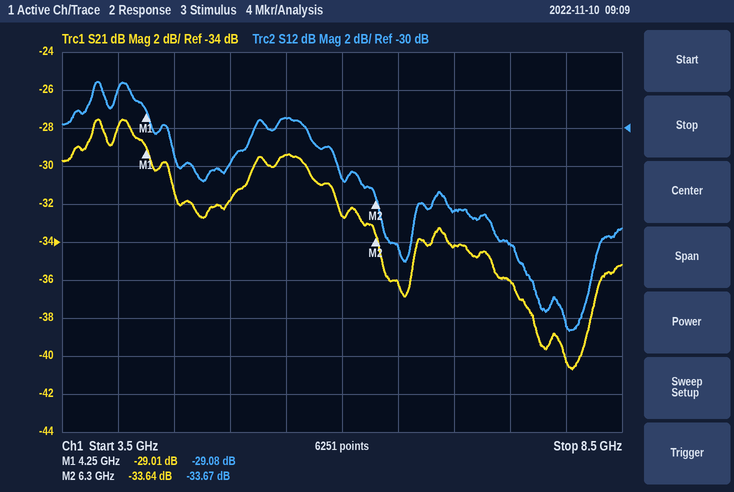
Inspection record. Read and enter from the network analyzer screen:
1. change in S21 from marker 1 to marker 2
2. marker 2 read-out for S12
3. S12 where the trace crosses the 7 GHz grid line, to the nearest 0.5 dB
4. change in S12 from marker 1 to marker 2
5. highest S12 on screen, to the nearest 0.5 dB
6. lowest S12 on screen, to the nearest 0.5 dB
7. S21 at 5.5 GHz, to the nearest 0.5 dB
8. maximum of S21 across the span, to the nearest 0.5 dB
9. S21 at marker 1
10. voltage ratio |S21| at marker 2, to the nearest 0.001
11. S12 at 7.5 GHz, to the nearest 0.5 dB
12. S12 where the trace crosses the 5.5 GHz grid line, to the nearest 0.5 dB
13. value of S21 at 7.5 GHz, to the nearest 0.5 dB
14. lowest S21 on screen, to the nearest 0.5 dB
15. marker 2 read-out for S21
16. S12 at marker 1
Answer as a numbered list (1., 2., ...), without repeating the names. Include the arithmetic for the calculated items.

1. -33.64 − (-29.01) = -4.63 dB
2. -33.67 dB
3. -34.5 dB
4. -33.67 − (-29.08) = -4.59 dB
5. -27.5 dB
6. -40.5 dB
7. -29.5 dB
8. -27.5 dB
9. -29.01 dB
10. 10^(-33.64/20) ≈ 0.021
11. -36.0 dB
12. -29.5 dB
13. -36.0 dB
14. -40.5 dB
15. -33.64 dB
16. -29.08 dB
